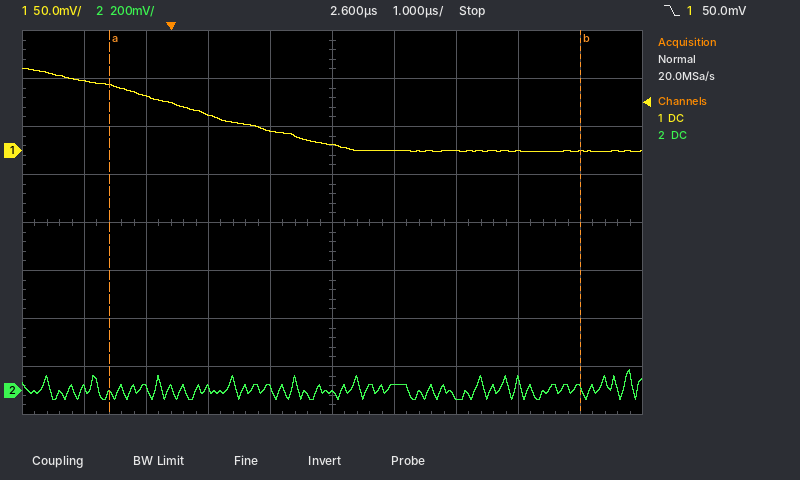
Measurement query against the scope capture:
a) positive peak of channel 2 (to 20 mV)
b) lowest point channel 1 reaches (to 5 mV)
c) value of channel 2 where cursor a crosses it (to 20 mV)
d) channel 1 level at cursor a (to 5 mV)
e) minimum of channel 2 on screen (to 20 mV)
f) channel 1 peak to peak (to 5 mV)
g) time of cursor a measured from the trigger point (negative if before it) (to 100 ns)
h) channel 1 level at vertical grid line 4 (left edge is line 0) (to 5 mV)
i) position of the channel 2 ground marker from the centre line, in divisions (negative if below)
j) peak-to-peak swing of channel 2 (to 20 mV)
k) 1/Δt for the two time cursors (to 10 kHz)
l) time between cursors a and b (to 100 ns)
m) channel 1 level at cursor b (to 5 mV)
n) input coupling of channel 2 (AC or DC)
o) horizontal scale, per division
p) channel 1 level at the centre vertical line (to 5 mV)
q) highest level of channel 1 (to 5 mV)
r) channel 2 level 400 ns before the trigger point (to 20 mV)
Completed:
80 mV
0 mV
-20 mV
70 mV
-40 mV
85 mV
-1.0 µs
20 mV
-3.5 div
120 mV
130 kHz
7.6 µs
0 mV
DC
1 µs
5 mV
85 mV
0 mV
